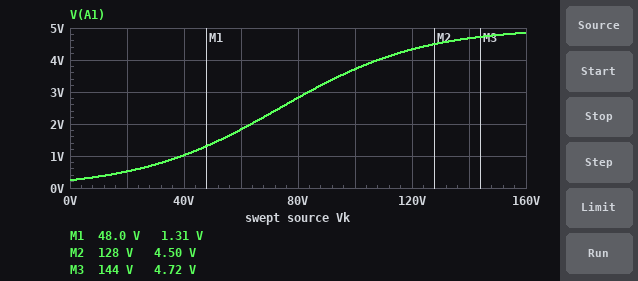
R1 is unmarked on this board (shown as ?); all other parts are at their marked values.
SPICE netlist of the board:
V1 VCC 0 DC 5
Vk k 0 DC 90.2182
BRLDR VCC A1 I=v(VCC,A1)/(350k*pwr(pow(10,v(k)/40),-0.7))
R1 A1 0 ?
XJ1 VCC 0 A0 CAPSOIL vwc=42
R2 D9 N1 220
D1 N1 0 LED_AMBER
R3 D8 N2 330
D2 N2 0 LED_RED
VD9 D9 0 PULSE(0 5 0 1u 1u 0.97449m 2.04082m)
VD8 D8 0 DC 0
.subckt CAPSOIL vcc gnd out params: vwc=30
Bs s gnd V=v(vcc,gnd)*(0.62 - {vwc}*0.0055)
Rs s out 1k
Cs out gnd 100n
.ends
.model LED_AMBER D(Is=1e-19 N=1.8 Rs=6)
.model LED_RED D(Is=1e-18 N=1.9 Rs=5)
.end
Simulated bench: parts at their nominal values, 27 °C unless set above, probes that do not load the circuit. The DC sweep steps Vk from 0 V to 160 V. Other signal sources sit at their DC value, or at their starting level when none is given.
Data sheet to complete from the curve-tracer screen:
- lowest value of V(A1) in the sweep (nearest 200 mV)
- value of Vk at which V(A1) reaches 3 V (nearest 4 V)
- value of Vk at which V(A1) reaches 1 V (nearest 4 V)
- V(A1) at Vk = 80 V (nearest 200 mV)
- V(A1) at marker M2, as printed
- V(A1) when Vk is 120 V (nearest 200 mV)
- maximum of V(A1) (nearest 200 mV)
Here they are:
200 mV
84 V
40 V
2.8 V
4.50 V
4.4 V
4.8 V
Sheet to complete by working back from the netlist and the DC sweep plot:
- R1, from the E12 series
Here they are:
18 kΩ
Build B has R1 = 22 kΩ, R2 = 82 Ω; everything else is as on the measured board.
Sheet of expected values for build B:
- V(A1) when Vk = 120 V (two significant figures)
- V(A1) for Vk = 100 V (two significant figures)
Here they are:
4.4 V
3.9 V
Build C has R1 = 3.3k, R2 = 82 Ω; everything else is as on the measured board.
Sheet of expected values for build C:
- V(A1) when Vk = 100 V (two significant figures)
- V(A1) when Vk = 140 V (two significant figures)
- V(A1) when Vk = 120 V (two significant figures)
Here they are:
1.7 V
3.6 V
2.7 V
